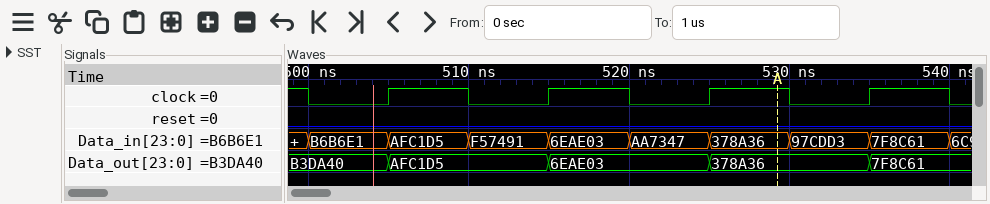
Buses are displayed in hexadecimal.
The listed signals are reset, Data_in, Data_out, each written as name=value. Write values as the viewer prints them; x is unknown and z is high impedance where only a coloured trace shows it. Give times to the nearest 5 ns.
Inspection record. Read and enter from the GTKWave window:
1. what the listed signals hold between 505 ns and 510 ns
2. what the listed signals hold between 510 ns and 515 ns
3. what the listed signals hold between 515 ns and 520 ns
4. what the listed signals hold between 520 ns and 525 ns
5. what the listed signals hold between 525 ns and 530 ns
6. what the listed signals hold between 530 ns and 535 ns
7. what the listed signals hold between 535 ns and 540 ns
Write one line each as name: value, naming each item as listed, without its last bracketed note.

what the listed signals hold between 505 ns and 510 ns: reset=0, Data_in=AFC1D5, Data_out=AFC1D5
what the listed signals hold between 510 ns and 515 ns: reset=0, Data_in=F57491, Data_out=AFC1D5
what the listed signals hold between 515 ns and 520 ns: reset=0, Data_in=6EAE03, Data_out=6EAE03
what the listed signals hold between 520 ns and 525 ns: reset=0, Data_in=AA7347, Data_out=6EAE03
what the listed signals hold between 525 ns and 530 ns: reset=0, Data_in=378A36, Data_out=378A36
what the listed signals hold between 530 ns and 535 ns: reset=0, Data_in=97CDD3, Data_out=378A36
what the listed signals hold between 535 ns and 540 ns: reset=0, Data_in=7F8C61, Data_out=7F8C61
